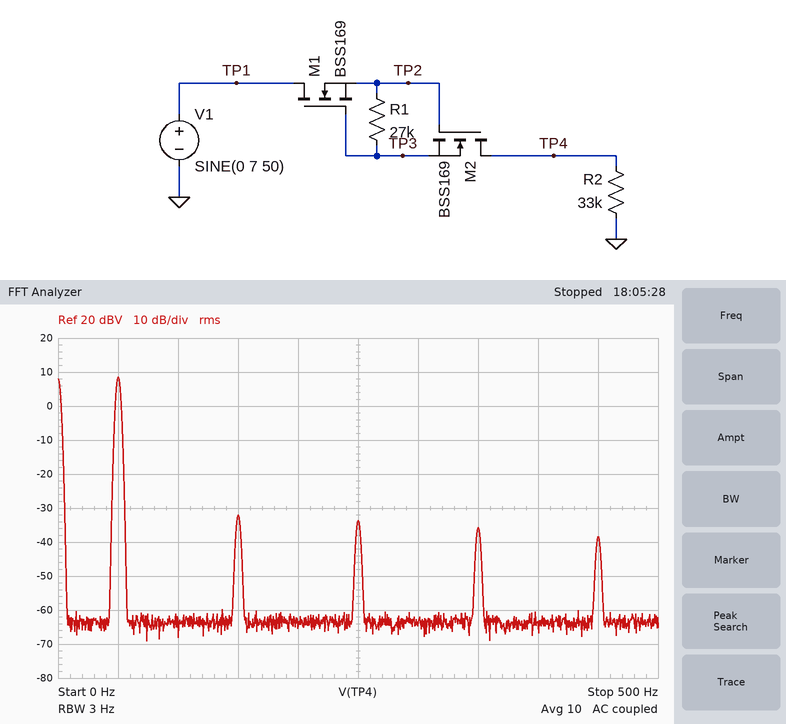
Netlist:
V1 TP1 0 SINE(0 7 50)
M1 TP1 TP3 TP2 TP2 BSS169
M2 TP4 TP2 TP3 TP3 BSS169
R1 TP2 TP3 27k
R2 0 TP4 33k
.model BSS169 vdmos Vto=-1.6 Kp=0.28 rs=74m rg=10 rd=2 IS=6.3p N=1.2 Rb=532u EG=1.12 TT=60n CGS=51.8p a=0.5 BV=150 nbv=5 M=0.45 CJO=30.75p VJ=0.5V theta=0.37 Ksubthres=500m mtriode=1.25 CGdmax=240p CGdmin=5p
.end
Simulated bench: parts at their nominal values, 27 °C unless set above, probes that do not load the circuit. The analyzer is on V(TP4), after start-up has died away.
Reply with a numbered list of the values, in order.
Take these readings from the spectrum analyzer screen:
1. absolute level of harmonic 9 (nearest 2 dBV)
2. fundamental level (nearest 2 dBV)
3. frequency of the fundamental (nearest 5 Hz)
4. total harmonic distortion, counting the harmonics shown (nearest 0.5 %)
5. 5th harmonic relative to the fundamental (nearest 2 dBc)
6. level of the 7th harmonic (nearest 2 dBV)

1. -38 dBV
2. 8 dBV
3. 50 Hz
4. 1.5 %
5. -42 dBc
6. -36 dBV
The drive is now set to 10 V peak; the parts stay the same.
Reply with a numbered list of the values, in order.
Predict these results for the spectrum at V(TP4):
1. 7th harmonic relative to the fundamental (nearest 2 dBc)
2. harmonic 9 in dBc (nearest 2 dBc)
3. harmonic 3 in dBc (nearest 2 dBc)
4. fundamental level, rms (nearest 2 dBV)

1. -32 dBc
2. -48 dBc
3. -16 dBc
4. 10 dBV
